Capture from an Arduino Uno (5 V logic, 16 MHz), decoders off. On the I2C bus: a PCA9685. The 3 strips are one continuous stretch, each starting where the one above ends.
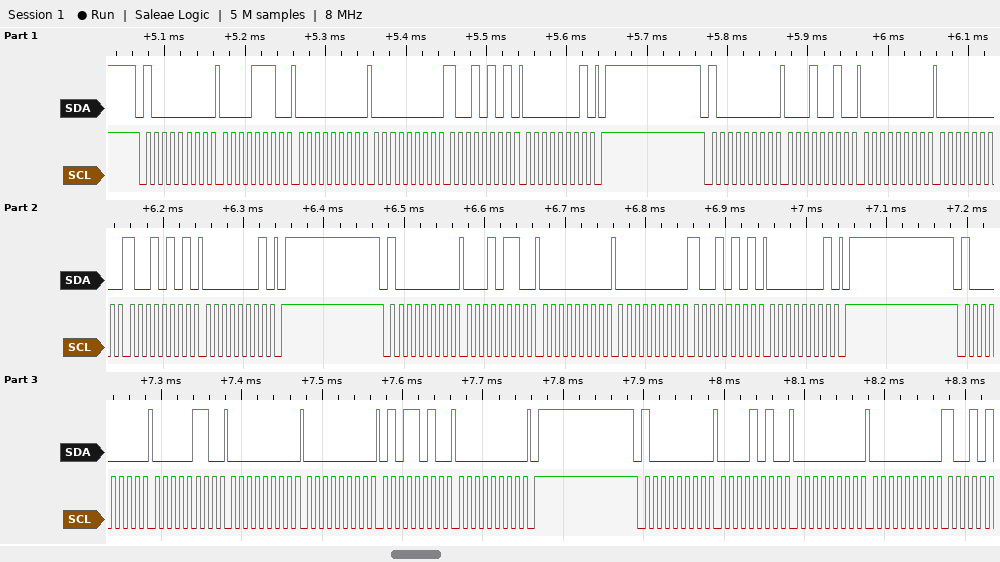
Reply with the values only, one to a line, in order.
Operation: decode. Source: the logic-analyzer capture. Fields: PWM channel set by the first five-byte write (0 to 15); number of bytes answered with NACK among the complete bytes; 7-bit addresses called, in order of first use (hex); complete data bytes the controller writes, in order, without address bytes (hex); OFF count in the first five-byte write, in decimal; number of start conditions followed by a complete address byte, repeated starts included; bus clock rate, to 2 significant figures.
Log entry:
2
0
0x40
0E 00 00 95 01 12 00 00 95 01 16 00 00 95 01 06 00 00 5A 00 0A 00 00
405
5
100 kHz
